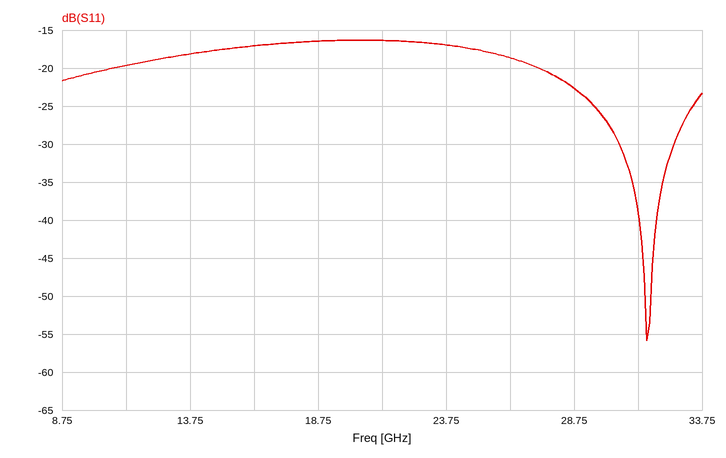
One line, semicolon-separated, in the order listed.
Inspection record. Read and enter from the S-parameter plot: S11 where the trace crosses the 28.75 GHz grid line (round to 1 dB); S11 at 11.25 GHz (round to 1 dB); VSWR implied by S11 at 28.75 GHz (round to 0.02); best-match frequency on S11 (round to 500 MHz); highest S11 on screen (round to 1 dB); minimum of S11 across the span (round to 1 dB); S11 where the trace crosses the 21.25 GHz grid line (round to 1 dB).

-23 dB; -20 dB; 1.16; 31.5 GHz; -16 dB; -56 dB; -16 dB
